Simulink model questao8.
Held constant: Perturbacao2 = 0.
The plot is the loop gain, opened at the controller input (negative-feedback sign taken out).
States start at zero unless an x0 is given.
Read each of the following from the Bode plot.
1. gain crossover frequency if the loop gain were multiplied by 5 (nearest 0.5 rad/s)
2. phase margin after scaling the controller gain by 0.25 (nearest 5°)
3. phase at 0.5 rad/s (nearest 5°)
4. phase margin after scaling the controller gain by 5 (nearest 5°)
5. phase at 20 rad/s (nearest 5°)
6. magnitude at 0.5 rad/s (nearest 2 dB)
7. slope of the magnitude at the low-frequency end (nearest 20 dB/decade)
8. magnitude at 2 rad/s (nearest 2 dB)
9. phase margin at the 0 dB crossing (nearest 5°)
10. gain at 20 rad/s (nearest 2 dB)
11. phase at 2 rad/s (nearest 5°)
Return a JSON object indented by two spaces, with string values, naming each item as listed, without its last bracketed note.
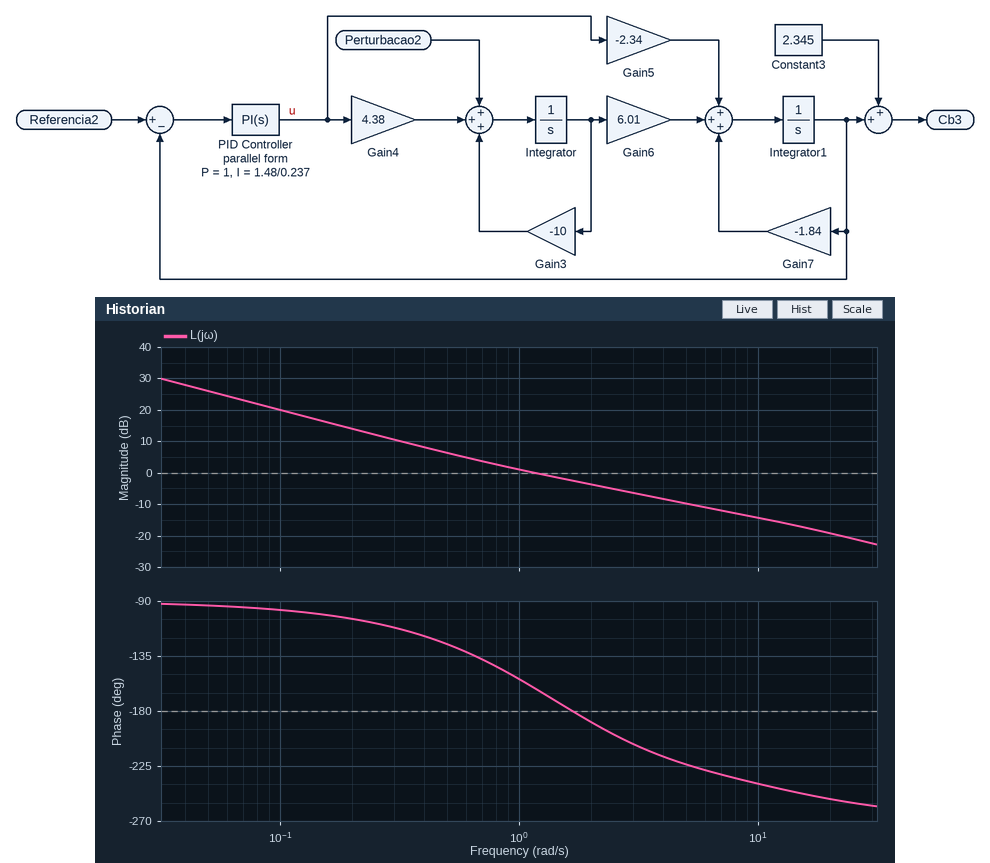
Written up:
{
  "gain crossover frequency if the loop gain were multiplied by 5": "9.5 rad/s",
  "phase margin after scaling the controller gain by 0.25": "70°",
  "phase at 0.5 rad/s": "-125°",
  "phase margin after scaling the controller gain by 5": "-60°",
  "phase at 20 rad/s": "-250°",
  "magnitude at 0.5 rad/s": "6 dB",
  "slope of the magnitude at the low-frequency end": "-20 dB/decade",
  "magnitude at 2 rad/s": "-4 dB",
  "phase margin at the 0 dB crossing": "20°",
  "gain at 20 rad/s": "-20 dB",
  "phase at 2 rad/s": "-190°"
}
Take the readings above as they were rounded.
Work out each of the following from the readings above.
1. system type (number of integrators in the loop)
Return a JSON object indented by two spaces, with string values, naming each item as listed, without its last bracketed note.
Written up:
{
  "system type": "1"
}
